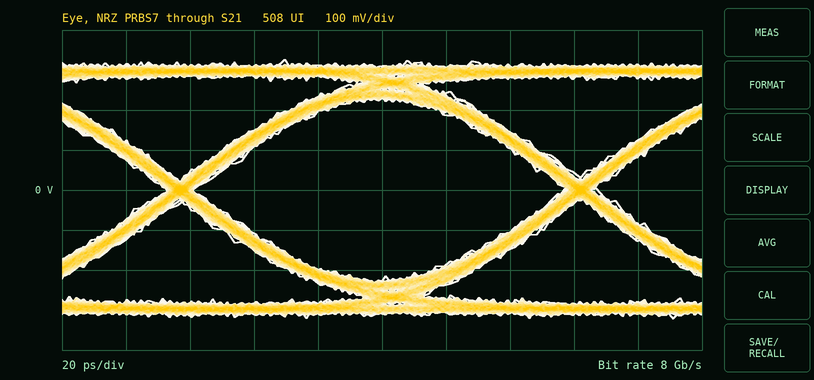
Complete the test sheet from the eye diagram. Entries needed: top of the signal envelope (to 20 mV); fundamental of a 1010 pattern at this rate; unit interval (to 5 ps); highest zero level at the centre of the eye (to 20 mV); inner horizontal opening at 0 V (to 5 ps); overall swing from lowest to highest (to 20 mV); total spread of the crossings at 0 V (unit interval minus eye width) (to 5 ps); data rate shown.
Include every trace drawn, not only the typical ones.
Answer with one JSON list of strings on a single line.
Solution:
["320 mV", "4 GHz", "125 ps", "-220 mV", "115 ps", "640 mV", "10 ps", "8 Gb/s"]
